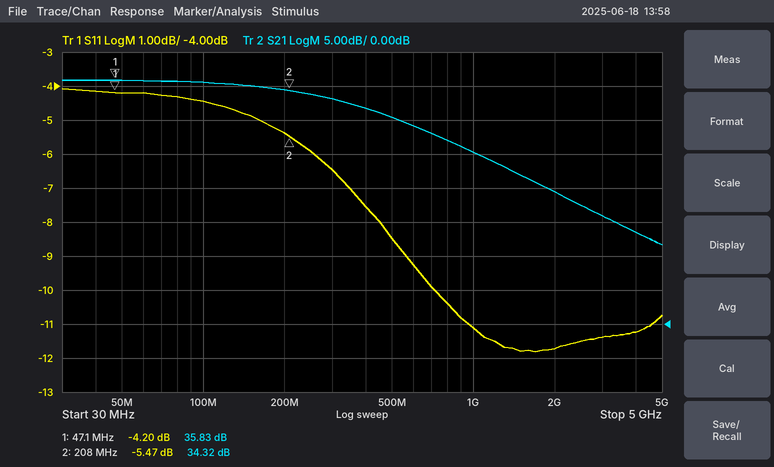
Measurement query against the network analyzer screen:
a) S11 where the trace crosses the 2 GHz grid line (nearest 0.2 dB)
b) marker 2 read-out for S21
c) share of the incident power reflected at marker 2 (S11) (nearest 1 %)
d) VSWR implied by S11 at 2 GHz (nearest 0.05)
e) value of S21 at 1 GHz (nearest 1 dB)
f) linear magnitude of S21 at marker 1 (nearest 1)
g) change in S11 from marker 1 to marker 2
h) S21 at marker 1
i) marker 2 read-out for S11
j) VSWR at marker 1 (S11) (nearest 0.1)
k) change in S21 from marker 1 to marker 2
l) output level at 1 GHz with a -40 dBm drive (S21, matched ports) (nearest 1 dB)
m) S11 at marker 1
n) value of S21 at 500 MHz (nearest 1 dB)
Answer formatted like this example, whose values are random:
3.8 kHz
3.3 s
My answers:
-11.8 dB
34.32 dB
28 %
1.70
25 dB
62
-1.27 dB
35.83 dB
-5.47 dB
4.2
-1.51 dB
-15 dBm
-4.20 dB
30 dB
